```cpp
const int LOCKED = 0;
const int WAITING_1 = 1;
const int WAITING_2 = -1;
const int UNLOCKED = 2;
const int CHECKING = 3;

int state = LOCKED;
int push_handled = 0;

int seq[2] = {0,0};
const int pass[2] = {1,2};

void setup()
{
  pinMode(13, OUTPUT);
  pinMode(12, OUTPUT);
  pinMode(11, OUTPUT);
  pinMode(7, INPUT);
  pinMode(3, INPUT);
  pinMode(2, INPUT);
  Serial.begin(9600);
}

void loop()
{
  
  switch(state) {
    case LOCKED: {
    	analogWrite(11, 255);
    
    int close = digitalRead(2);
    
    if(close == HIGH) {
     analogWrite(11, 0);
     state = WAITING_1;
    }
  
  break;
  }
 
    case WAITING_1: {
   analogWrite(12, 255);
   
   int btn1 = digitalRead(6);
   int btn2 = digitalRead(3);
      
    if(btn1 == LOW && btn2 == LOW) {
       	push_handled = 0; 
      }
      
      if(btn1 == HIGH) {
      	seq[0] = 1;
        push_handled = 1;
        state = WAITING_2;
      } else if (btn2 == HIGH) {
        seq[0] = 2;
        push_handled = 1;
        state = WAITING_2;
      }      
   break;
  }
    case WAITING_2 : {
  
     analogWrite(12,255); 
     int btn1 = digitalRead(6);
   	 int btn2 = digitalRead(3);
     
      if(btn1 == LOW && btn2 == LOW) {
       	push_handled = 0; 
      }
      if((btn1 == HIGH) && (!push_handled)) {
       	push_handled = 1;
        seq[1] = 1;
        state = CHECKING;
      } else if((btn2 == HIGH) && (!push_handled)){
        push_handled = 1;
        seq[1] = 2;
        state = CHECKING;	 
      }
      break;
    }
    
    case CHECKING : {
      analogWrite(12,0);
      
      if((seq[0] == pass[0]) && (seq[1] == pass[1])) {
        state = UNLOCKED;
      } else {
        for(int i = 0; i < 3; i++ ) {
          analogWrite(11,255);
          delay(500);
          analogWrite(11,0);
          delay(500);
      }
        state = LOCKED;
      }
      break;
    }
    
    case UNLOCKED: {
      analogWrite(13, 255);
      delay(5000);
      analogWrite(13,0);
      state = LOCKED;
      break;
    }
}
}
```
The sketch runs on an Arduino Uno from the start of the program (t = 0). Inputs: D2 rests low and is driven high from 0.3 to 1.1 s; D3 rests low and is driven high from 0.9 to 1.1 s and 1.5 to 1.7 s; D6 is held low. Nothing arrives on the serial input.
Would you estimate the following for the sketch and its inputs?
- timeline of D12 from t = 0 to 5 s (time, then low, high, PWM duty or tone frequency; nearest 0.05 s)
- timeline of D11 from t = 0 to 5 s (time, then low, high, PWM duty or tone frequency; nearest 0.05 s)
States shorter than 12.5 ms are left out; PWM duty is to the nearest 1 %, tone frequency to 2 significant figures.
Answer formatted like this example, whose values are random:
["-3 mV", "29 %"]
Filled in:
["0 s low; 0.3 s high; 1.5 s low", "0 s high; 0.3 s low; 1.5 s high; 2 s low; 2.5 s high; 3 s low; 3.5 s high; 4 s low; 4.5 s high"]
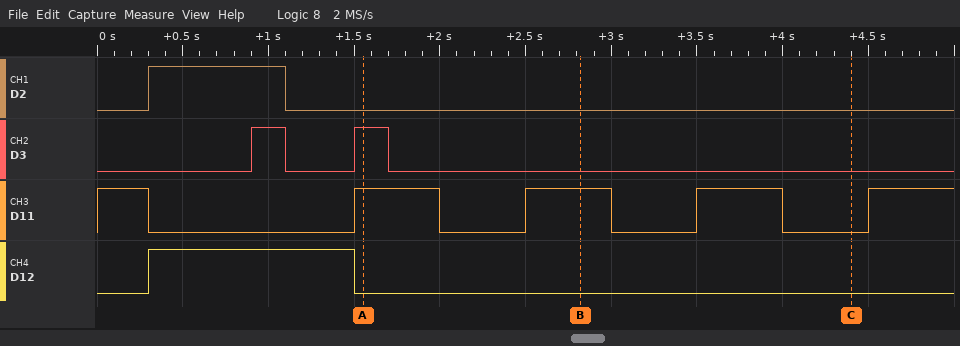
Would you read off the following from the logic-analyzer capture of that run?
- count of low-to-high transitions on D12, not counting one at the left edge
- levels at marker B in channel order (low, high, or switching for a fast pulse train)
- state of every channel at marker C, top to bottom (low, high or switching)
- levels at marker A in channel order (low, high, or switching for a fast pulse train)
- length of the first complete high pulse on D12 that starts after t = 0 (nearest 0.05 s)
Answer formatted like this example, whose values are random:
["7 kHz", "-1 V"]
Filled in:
["1", "D2 low, D3 low, D11 high, D12 low", "D2 low, D3 low, D11 low, D12 low", "D2 low, D3 high, D11 high, D12 low", "1.20 s"]
